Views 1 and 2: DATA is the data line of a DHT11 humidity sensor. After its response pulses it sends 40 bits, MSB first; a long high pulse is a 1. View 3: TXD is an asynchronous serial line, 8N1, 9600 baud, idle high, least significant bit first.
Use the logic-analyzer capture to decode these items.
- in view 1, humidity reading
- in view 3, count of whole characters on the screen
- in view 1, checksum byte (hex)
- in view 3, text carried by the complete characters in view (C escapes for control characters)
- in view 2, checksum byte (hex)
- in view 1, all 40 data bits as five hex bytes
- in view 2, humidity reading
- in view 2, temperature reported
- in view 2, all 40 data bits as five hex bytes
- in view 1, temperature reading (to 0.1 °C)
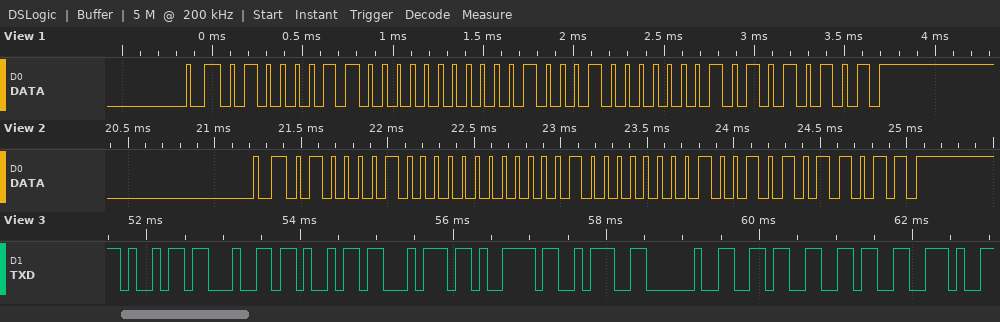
67 %
10
0x55
"idity: 66."
0x5B
43 00 11 01 55
66 %
16.9 °C
42 00 10 09 5B
17.1 °C
